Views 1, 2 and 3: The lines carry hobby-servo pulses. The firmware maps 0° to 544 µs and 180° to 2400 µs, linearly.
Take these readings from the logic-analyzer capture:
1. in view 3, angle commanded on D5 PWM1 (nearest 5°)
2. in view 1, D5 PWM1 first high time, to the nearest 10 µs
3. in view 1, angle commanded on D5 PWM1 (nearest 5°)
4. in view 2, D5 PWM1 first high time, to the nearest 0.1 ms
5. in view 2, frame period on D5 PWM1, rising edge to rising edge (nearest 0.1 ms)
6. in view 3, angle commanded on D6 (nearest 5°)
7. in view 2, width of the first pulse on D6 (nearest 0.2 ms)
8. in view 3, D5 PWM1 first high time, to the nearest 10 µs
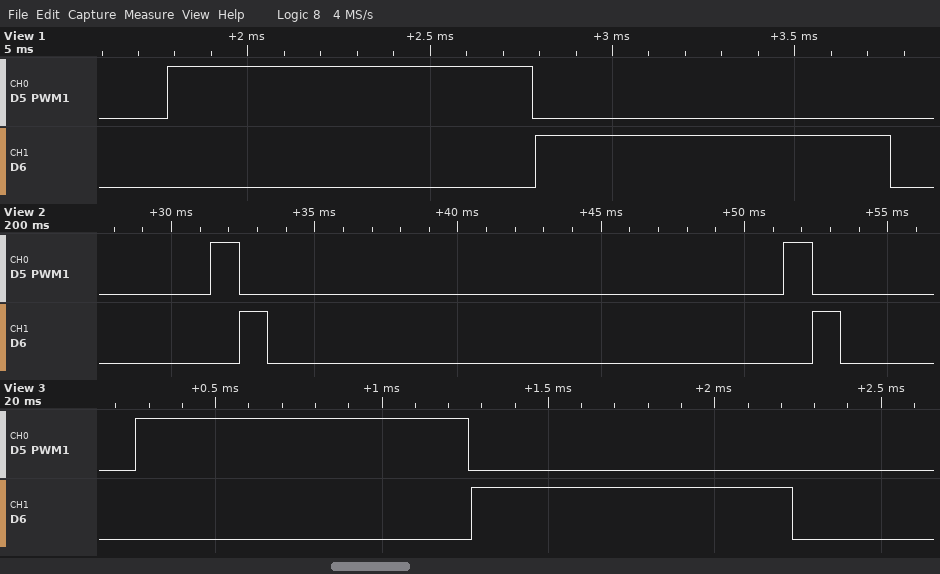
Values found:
45°
1000 µs
45°
1.0 ms
20.0 ms
40°
1.0 ms
1000 µs
